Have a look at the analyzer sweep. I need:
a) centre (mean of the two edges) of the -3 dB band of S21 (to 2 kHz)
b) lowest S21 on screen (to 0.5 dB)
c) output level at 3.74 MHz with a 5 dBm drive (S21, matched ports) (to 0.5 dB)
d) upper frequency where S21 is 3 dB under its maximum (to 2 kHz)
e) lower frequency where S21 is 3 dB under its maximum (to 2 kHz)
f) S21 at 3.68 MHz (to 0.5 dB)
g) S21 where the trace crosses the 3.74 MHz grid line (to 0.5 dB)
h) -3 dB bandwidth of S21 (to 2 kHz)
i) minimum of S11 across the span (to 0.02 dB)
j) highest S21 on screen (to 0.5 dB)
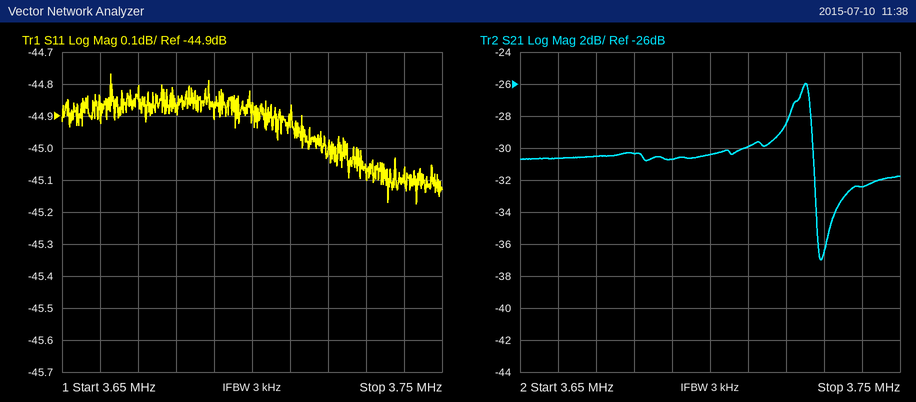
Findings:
3.722 MHz
-37.0 dB
-27.5 dBm
3.726 MHz
3.718 MHz
-30.5 dB
-32.5 dB
8 kHz
-45.18 dB
-26.0 dB
